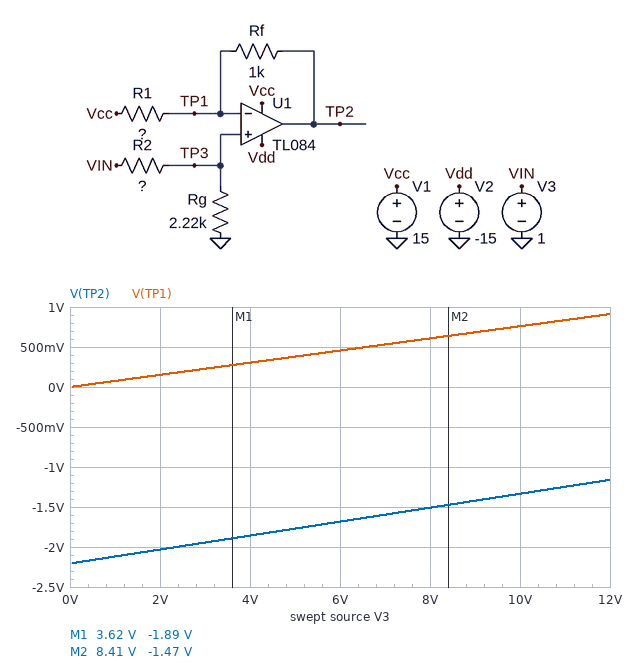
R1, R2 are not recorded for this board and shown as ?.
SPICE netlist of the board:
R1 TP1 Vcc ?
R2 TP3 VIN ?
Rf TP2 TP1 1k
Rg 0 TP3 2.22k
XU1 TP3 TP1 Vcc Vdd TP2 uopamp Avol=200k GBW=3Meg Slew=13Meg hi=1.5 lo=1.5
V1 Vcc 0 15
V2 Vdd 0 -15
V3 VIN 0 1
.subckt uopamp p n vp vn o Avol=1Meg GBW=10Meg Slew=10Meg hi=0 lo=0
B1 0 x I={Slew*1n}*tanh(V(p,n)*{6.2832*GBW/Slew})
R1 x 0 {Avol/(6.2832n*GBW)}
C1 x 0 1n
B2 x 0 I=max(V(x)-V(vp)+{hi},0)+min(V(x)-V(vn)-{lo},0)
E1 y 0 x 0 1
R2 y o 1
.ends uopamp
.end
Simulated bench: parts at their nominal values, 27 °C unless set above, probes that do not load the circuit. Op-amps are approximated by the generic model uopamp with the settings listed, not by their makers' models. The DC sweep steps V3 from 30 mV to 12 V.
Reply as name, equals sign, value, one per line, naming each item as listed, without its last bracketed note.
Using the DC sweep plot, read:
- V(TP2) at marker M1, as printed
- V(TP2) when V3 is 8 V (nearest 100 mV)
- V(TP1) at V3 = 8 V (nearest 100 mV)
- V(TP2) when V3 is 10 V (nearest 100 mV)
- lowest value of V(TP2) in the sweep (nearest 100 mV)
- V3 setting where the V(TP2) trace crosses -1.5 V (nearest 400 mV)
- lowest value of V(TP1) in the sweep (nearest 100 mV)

V(TP2) at marker M1, as printed = -1.89 V
V(TP2) when V3 is 8 V = -1.5 V
V(TP1) at V3 = 8 V = 600 mV
V(TP2) when V3 is 10 V = -1.3 V
lowest value of V(TP2) in the sweep = -2.2 V
V3 setting where the V(TP2) trace crosses -1.5 V = 8.0 V
lowest value of V(TP1) in the sweep = 0 V
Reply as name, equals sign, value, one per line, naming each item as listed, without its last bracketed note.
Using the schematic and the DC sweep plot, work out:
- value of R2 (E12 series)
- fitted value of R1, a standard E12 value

value of R2 = 27 kΩ
fitted value of R1, a standard E12 value = 6.8 kΩ
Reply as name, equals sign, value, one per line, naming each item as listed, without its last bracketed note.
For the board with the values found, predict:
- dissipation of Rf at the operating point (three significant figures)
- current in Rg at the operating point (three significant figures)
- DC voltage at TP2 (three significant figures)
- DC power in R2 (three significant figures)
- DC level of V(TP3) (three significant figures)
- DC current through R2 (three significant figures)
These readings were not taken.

dissipation of Rf at the operating point = 4.82 mW
current in Rg at the operating point = 34.2 µA
DC voltage at TP2 = -2.12 V
DC power in R2 = 31.6 µW
DC level of V(TP3) = 76.0 mV
DC current through R2 = 34.2 µA
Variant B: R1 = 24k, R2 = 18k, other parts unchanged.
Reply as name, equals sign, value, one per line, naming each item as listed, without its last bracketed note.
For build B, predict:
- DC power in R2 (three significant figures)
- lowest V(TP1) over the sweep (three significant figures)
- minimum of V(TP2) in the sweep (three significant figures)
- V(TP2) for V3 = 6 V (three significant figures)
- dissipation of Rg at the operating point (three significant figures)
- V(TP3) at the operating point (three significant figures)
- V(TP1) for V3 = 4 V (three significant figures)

DC power in R2 = 44.0 µW
lowest V(TP1) over the sweep = 3.30 mV
minimum of V(TP2) in the sweep = -622 mV
V(TP2) for V3 = 6 V = 61.2 mV
dissipation of Rg at the operating point = 5.43 µW
V(TP3) at the operating point = 110 mV
V(TP1) for V3 = 4 V = 439 mV
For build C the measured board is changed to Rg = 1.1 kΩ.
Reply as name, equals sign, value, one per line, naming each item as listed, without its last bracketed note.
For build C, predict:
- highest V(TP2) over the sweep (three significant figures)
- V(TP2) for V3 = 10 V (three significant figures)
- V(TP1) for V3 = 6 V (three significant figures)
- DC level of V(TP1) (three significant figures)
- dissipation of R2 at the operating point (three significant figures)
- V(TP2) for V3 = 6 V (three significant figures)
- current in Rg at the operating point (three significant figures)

highest V(TP2) over the sweep = -1.67 V
V(TP2) for V3 = 10 V = -1.76 V
V(TP1) for V3 = 6 V = 235 mV
DC level of V(TP1) = 39.2 mV
dissipation of R2 at the operating point = 34.2 µW
V(TP2) for V3 = 6 V = -1.94 V
current in Rg at the operating point = 35.6 µA
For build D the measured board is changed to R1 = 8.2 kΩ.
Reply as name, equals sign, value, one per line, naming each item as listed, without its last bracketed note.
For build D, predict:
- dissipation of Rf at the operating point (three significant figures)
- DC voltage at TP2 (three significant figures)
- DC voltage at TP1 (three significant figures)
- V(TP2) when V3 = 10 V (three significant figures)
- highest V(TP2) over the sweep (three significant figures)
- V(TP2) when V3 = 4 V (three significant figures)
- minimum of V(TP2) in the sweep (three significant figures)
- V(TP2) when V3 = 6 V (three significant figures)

dissipation of Rf at the operating point = 3.31 mW
DC voltage at TP2 = -1.74 V
DC voltage at TP1 = 76.0 mV
V(TP2) when V3 = 10 V = -977 mV
highest V(TP2) over the sweep = -806 mV
V(TP2) when V3 = 4 V = -1.49 V
minimum of V(TP2) in the sweep = -1.83 V
V(TP2) when V3 = 6 V = -1.32 V
